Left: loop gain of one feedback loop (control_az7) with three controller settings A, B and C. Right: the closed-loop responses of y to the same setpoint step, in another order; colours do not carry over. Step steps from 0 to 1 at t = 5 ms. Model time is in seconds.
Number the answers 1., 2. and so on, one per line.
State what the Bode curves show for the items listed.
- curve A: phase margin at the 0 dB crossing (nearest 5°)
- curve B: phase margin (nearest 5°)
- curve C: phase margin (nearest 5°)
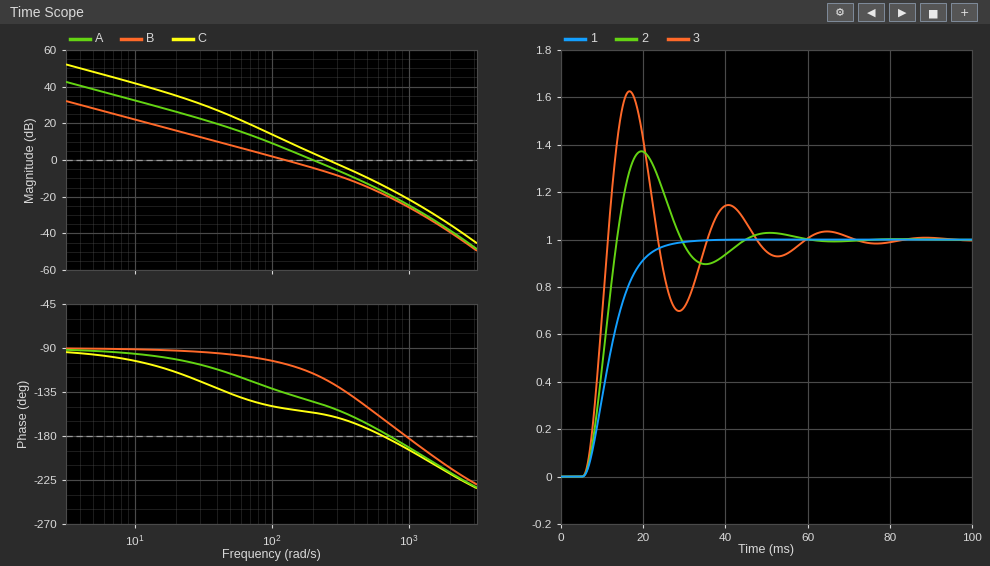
1. 35°
2. 75°
3. 20°
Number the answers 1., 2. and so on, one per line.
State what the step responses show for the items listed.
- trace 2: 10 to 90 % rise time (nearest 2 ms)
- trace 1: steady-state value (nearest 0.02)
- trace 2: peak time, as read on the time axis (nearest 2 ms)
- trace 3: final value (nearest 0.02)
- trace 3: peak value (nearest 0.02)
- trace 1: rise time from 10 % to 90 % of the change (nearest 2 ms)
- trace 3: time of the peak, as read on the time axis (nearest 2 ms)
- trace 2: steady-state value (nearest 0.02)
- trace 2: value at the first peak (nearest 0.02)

1. 6 ms
2. 1.00
3. 20 ms
4. 1.00
5. 1.62
6. 12 ms
7. 16 ms
8. 1.00
9. 1.38
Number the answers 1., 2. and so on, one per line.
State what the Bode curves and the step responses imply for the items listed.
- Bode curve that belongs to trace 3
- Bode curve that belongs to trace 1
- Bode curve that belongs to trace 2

1. C
2. B
3. A
